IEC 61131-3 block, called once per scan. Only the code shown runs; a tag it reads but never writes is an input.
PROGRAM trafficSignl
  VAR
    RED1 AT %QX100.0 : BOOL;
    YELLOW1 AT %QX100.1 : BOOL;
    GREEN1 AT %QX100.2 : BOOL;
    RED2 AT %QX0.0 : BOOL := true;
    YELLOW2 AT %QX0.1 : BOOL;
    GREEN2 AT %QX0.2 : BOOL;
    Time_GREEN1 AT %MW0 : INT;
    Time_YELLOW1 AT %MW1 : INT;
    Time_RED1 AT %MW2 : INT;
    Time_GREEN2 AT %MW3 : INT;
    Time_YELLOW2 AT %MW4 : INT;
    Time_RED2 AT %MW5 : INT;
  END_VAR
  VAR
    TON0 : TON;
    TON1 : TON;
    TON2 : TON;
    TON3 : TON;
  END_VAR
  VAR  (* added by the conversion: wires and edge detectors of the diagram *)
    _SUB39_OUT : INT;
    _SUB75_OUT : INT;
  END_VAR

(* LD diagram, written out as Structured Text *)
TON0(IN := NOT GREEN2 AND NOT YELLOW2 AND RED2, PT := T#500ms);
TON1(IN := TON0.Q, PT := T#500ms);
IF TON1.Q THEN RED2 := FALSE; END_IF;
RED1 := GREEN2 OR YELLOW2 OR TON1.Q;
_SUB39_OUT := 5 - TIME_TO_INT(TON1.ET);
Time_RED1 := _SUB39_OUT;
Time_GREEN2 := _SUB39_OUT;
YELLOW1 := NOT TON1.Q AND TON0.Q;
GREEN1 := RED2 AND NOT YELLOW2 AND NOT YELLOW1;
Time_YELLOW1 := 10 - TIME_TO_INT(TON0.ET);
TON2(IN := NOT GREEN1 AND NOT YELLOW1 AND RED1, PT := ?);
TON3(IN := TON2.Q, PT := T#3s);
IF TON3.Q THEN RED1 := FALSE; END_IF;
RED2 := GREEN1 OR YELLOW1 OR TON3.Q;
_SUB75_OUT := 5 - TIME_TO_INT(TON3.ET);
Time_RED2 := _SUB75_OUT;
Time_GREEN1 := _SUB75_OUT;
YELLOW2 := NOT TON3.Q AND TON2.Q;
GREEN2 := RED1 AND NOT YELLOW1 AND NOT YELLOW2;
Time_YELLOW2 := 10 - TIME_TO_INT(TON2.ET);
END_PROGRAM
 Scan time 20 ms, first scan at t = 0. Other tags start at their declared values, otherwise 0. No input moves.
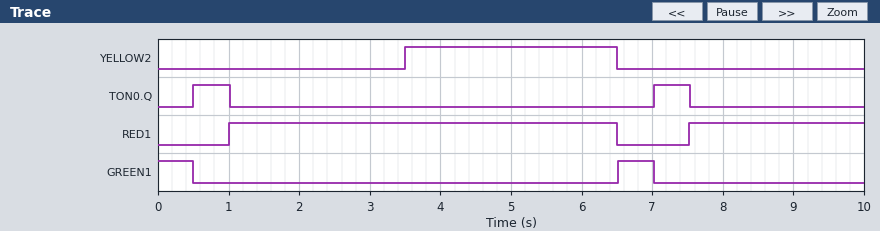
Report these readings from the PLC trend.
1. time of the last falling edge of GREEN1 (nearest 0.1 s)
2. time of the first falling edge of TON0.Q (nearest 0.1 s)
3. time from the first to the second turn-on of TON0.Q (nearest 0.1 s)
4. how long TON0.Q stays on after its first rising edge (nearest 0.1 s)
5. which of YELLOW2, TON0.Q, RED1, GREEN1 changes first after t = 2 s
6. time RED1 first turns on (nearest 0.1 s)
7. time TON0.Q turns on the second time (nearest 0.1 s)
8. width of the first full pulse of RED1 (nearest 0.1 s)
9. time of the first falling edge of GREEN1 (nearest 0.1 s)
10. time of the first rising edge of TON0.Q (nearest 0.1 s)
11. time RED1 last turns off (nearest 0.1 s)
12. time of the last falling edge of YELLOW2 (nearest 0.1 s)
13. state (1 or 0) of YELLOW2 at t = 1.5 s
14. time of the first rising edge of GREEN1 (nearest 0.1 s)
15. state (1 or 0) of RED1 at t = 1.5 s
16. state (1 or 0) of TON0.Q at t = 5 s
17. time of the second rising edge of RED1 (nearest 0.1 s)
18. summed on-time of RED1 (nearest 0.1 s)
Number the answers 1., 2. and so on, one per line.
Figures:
1. 7.0 s
2. 1.0 s
3. 6.5 s
4. 0.5 s
5. YELLOW2
6. 1.0 s
7. 7.0 s
8. 5.5 s
9. 0.5 s
10. 0.5 s
11. 6.5 s
12. 6.5 s
13. 0
14. 6.5 s
15. 1
16. 0
17. 7.5 s
18. 8.0 s
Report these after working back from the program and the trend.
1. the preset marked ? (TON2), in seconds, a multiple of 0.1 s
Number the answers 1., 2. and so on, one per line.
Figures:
1. 2.5 s
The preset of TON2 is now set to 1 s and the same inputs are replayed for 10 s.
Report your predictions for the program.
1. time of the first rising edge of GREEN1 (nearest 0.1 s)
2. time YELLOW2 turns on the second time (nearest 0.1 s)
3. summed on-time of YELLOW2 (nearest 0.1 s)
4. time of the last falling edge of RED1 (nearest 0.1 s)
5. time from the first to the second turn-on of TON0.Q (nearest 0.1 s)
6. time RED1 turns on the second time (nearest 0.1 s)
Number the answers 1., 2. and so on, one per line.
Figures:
1. 5.0 s
2. 7.0 s
3. 6.0 s
4. 5.0 s
5. 5.0 s
6. 6.0 s
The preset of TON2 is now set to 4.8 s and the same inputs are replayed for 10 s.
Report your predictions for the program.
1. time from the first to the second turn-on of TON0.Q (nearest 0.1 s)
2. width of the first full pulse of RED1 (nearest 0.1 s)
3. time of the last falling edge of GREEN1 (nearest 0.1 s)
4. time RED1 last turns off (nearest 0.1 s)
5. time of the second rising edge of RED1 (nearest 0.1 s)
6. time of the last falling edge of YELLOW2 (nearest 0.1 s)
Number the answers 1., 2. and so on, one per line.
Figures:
1. 8.8 s
2. 7.8 s
3. 9.3 s
4. 8.8 s
5. 9.8 s
6. 8.8 s
